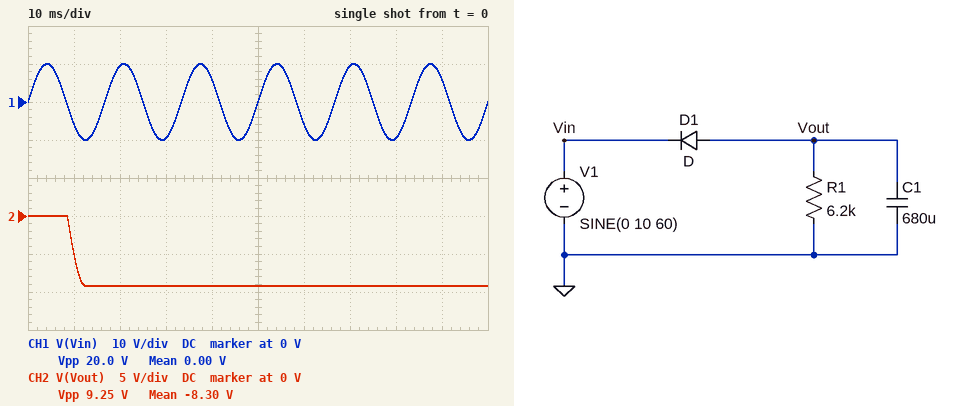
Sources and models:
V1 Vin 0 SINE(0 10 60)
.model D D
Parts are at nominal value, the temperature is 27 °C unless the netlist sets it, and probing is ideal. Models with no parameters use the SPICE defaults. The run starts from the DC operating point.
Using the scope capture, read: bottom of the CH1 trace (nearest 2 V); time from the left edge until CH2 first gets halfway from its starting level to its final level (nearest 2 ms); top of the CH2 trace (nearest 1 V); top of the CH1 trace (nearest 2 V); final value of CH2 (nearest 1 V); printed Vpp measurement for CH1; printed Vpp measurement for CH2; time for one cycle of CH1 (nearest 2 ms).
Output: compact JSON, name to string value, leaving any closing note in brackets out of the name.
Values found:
{"bottom of the CH1 trace": "-10 V", "time from the left edge until CH2 first gets halfway from its starting level to its final level": "10 ms", "top of the CH2 trace": "0 V", "top of the CH1 trace": "10 V", "final value of CH2": "-9 V", "printed Vpp measurement for CH1": "20.0 V", "printed Vpp measurement for CH2": "9.25 V", "time for one cycle of CH1": "16 ms"}
